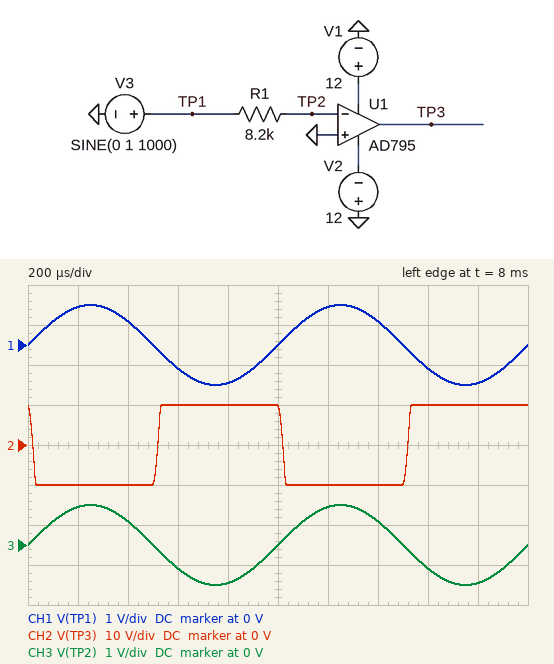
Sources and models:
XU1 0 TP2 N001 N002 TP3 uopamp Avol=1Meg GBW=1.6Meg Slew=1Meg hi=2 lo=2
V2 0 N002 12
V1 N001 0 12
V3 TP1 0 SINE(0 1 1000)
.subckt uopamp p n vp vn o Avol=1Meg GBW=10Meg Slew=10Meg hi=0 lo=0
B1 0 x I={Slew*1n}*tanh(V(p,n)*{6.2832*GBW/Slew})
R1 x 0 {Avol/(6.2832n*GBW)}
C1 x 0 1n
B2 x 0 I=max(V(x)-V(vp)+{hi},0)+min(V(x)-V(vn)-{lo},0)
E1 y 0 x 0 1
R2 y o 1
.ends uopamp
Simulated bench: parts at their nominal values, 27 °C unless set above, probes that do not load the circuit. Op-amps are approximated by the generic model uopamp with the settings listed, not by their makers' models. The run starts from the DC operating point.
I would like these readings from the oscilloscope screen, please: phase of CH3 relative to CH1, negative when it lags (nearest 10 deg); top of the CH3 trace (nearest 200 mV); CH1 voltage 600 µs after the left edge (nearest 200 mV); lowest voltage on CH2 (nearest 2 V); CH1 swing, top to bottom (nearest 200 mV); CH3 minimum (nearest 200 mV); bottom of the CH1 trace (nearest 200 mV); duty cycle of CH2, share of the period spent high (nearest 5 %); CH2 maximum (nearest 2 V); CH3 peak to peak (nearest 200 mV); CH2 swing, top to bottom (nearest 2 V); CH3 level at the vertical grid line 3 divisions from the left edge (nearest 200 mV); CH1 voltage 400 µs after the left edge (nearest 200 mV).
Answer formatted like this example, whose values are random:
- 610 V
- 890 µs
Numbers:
- 0 deg
- 1.0 V
- -600 mV
- -10 V
- 2.0 V
- -1.0 V
- -1.0 V
- 50 %
- 10 V
- 2.0 V
- 20 V
- -600 mV
- 600 mV
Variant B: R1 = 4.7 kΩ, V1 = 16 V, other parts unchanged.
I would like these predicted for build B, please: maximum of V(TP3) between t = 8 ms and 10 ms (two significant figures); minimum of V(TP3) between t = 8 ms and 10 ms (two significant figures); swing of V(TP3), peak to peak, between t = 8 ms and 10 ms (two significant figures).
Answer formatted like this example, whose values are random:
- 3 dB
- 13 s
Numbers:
- 14 V
- -10 V
- 24 V
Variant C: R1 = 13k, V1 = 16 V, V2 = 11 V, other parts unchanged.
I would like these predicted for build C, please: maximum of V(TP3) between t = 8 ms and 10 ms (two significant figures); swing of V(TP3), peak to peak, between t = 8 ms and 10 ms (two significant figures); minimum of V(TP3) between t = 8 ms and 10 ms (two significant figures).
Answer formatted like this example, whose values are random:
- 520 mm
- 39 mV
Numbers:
- 14 V
- 23 V
- -9.0 V
